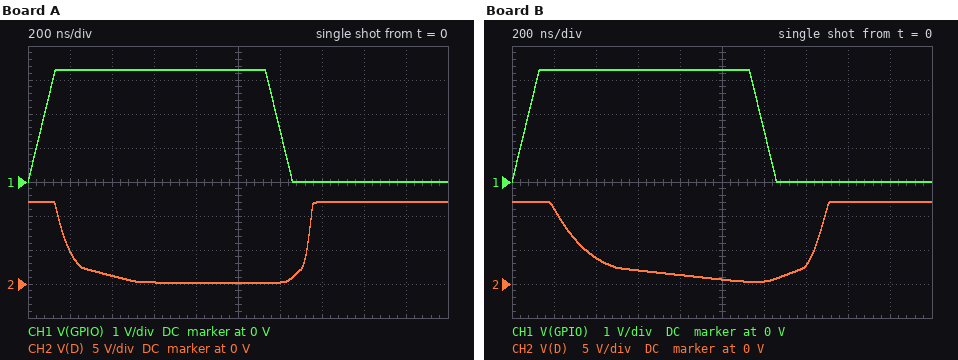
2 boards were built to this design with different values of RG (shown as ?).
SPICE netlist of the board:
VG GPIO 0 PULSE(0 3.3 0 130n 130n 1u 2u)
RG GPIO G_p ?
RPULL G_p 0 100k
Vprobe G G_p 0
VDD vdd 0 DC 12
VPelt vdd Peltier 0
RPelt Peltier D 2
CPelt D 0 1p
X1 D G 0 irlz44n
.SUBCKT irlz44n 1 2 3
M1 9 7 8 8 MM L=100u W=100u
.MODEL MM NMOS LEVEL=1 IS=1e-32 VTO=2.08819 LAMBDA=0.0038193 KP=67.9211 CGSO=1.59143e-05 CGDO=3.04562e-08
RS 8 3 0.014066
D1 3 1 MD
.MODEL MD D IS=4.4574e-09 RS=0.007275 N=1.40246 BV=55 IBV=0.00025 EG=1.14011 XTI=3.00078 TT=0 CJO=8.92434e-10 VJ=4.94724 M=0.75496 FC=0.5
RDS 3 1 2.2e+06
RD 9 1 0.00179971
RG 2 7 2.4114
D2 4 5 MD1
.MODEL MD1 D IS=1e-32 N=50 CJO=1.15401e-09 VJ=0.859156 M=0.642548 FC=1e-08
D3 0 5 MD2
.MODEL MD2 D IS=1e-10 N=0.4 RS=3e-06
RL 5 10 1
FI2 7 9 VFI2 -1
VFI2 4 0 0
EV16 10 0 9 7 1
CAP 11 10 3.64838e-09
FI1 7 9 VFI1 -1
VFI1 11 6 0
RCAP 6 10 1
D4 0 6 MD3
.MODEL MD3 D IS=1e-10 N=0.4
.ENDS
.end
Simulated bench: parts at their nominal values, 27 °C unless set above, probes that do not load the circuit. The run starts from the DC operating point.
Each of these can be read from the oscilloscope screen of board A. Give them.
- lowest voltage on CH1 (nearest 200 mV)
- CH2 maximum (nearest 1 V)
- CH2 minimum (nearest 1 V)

0 V
12 V
0 V
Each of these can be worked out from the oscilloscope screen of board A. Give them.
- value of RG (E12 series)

22 Ω
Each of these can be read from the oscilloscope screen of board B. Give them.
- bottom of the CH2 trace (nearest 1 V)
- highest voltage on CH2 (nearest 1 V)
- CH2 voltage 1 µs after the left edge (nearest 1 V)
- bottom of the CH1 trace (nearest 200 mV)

0 V
12 V
1 V
0 V
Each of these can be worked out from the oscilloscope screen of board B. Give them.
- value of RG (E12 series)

56 Ω
